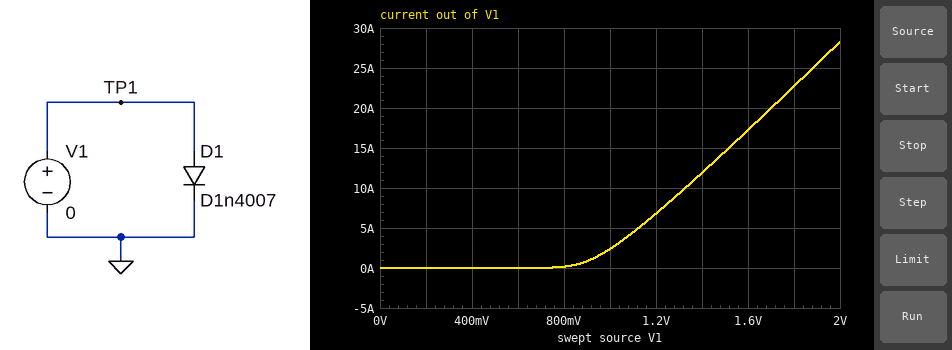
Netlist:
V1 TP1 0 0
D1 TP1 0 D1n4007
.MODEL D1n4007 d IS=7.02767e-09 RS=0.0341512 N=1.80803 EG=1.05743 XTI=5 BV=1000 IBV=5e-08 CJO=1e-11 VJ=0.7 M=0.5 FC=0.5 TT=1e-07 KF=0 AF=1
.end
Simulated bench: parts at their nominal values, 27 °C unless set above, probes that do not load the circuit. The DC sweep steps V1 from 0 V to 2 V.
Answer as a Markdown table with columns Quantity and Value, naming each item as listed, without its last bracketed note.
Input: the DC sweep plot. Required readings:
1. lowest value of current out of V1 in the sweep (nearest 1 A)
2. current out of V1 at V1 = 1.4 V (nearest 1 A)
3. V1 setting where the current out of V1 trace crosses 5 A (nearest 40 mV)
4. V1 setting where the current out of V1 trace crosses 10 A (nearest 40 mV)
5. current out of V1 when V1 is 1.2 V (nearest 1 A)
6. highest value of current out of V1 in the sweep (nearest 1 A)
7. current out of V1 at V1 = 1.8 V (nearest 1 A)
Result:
| Quantity | Value |
|---|---|
| lowest value of current out of V1 in the sweep | 0 A |
| current out of V1 at V1 = 1.4 V | 12 A |
| V1 setting where the current out of V1 trace crosses 5 A | 1.12 V |
| V1 setting where the current out of V1 trace crosses 10 A | 1.32 V |
| current out of V1 when V1 is 1.2 V | 7 A |
| highest value of current out of V1 in the sweep | 28 A |
| current out of V1 at V1 = 1.8 V | 23 A |
